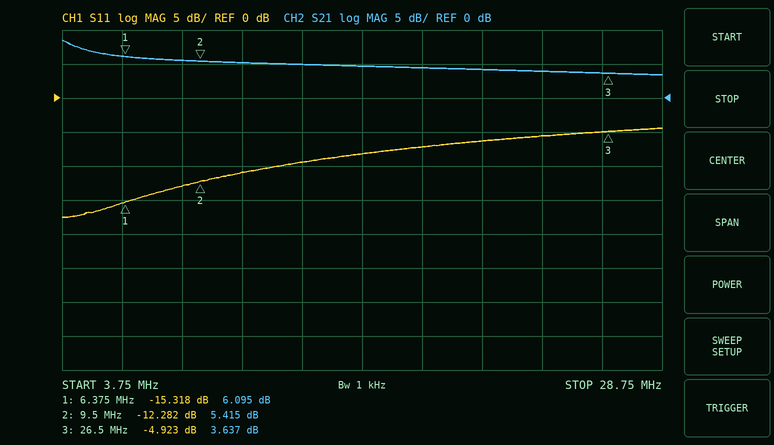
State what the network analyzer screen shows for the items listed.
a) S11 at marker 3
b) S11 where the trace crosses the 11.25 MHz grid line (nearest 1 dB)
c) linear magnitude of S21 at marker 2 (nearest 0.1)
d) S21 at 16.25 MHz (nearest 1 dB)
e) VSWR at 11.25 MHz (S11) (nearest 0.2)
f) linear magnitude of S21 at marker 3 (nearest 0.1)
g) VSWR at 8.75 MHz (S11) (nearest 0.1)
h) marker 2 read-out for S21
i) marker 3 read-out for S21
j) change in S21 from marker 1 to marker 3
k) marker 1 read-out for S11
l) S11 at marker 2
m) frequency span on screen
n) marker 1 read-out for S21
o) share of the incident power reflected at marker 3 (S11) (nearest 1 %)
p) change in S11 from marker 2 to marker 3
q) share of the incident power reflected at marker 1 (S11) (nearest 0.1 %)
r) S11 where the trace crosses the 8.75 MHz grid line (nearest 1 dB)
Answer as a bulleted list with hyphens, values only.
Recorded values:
- -4.923 dB
- -11 dB
- 1.9
- 5 dB
- 1.8
- 1.5
- 1.6
- 5.415 dB
- 3.637 dB
- -2.458 dB
- -15.318 dB
- -12.282 dB
- 25 MHz
- 6.095 dB
- 32 %
- 7.359 dB
- 2.9 %
- -13 dB
